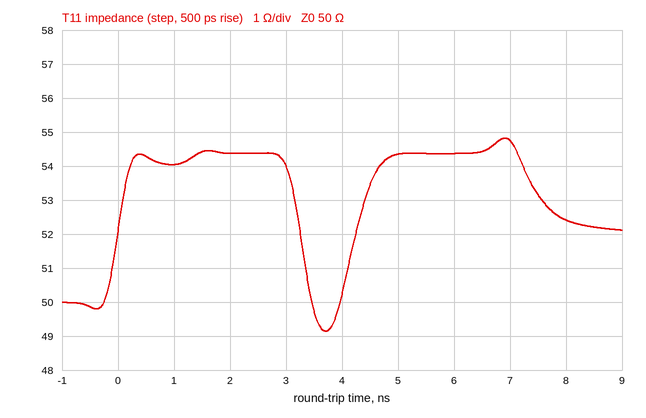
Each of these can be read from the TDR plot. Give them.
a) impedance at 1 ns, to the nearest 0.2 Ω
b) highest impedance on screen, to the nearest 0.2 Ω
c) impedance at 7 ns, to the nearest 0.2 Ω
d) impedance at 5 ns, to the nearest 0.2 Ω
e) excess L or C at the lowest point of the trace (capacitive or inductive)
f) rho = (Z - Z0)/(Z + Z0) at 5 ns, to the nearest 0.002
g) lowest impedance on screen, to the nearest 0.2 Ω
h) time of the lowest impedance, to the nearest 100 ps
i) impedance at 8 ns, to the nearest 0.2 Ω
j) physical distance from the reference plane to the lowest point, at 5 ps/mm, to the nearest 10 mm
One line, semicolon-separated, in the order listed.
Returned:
54.0 Ω; 54.8 Ω; 54.8 Ω; 54.4 Ω; capacitive; +0.042; 49.2 Ω; 3.7 ns; 52.4 Ω; 370 mm
